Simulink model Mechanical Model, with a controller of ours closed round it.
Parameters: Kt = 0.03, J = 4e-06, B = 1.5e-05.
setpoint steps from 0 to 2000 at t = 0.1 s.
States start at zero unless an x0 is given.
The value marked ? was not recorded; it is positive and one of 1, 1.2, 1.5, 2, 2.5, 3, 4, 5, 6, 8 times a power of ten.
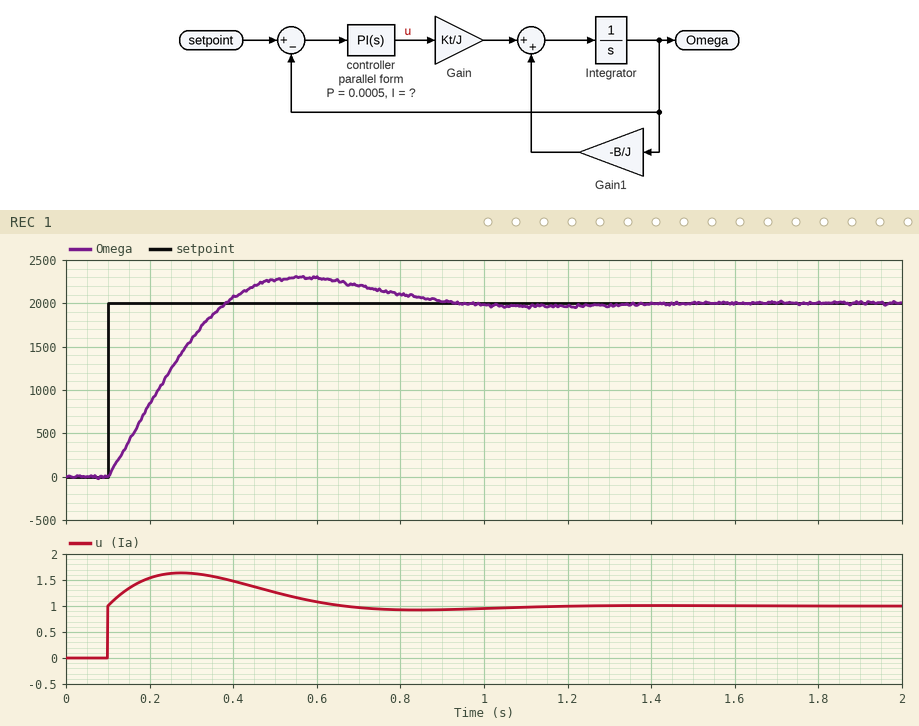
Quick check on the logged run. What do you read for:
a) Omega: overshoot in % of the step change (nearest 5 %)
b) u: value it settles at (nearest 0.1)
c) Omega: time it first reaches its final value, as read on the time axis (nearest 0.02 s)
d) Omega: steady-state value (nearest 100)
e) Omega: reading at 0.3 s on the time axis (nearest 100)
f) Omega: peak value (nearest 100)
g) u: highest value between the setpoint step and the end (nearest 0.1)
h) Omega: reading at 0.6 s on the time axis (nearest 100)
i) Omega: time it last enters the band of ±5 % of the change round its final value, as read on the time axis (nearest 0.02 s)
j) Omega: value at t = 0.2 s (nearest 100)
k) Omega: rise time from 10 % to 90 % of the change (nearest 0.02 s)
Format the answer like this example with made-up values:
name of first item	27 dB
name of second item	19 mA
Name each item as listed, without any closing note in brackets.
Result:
Omega: overshoot in % of the step change	15 %
u: value it settles at	1.0
Omega: time it first reaches its final value, as read on the time axis	0.38 s
Omega: steady-state value	2000
Omega: reading at 0.3 s on the time axis	1600
Omega: peak value	2300
u: highest value between the setpoint step and the end	1.6
Omega: reading at 0.6 s on the time axis	2300
Omega: time it last enters the band of ±5 % of the change round its final value, as read on the time axis	0.80 s
Omega: value at t = 0.2 s	800
Omega: rise time from 10 % to 90 % of the change	0.22 s
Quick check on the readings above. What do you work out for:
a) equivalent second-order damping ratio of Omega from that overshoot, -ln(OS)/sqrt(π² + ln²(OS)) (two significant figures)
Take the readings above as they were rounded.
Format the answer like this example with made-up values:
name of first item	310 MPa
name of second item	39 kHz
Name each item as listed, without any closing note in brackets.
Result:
equivalent second-order damping ratio of Omega from that overshoot, -ln(OS)/sqrt(π² + ln²(OS))	0.52
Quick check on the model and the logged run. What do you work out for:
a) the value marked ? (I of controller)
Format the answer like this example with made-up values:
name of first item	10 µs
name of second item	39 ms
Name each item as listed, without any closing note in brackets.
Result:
the value marked ?	0.006
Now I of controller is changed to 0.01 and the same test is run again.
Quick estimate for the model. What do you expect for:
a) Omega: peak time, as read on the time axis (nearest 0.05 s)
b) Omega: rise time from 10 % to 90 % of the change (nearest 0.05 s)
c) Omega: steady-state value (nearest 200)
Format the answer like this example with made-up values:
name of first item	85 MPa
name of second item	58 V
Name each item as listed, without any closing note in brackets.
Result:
Omega: peak time, as read on the time axis	0.45 s
Omega: rise time from 10 % to 90 % of the change	0.15 s
Omega: steady-state value	2000
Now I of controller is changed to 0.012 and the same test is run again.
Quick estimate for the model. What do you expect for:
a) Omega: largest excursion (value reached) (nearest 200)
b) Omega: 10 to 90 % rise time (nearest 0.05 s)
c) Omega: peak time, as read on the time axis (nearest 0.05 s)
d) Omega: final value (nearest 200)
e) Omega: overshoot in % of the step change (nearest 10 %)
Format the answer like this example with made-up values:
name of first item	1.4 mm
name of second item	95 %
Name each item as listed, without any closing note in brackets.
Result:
Omega: largest excursion (value reached)	2600
Omega: 10 to 90 % rise time	0.15 s
Omega: peak time, as read on the time axis	0.40 s
Omega: final value	2000
Omega: overshoot in % of the step change	30 %
